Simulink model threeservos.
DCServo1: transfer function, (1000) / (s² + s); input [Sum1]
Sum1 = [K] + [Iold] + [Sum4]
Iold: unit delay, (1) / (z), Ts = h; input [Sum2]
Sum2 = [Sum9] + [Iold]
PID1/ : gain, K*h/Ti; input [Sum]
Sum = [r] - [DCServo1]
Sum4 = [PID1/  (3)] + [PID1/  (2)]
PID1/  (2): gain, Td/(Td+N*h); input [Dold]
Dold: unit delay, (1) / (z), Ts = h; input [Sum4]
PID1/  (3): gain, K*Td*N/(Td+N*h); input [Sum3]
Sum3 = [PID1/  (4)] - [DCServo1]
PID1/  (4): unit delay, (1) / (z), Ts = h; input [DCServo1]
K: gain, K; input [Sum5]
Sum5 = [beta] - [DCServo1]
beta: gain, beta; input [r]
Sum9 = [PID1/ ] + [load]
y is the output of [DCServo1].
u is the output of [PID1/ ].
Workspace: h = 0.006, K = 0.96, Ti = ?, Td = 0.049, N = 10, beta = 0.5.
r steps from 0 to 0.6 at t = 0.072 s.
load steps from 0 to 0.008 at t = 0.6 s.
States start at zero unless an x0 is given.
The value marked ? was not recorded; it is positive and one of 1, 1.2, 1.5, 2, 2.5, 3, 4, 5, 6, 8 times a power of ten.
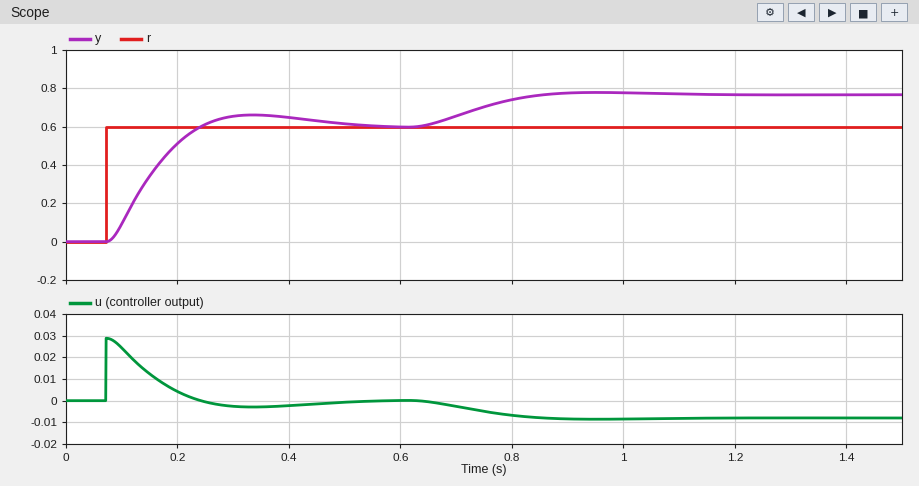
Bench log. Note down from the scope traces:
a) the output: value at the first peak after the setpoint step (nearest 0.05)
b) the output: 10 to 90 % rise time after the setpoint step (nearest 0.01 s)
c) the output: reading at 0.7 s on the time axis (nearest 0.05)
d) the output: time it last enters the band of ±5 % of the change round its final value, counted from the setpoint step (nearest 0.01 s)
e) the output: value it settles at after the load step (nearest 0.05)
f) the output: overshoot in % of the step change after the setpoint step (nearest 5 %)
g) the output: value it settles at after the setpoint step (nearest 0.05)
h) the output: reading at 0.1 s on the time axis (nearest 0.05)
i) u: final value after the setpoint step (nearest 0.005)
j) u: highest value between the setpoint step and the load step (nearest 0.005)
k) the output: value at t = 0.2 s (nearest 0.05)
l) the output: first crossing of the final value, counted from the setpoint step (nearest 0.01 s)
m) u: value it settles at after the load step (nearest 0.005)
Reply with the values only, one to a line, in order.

0.65
0.12 s
0.65
0.38 s
0.75
10 %
0.60
0.10
0.000
0.030
0.50
0.17 s
-0.010
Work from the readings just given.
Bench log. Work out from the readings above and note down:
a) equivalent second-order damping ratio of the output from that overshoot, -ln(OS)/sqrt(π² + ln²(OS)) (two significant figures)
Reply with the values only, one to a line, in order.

0.59
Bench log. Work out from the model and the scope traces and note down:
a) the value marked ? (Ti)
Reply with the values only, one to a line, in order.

0.12
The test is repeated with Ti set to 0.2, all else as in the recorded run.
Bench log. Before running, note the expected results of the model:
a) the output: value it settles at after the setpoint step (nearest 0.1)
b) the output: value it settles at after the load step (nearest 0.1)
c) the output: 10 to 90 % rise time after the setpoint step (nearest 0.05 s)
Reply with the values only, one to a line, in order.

0.6
0.9
0.20 s
